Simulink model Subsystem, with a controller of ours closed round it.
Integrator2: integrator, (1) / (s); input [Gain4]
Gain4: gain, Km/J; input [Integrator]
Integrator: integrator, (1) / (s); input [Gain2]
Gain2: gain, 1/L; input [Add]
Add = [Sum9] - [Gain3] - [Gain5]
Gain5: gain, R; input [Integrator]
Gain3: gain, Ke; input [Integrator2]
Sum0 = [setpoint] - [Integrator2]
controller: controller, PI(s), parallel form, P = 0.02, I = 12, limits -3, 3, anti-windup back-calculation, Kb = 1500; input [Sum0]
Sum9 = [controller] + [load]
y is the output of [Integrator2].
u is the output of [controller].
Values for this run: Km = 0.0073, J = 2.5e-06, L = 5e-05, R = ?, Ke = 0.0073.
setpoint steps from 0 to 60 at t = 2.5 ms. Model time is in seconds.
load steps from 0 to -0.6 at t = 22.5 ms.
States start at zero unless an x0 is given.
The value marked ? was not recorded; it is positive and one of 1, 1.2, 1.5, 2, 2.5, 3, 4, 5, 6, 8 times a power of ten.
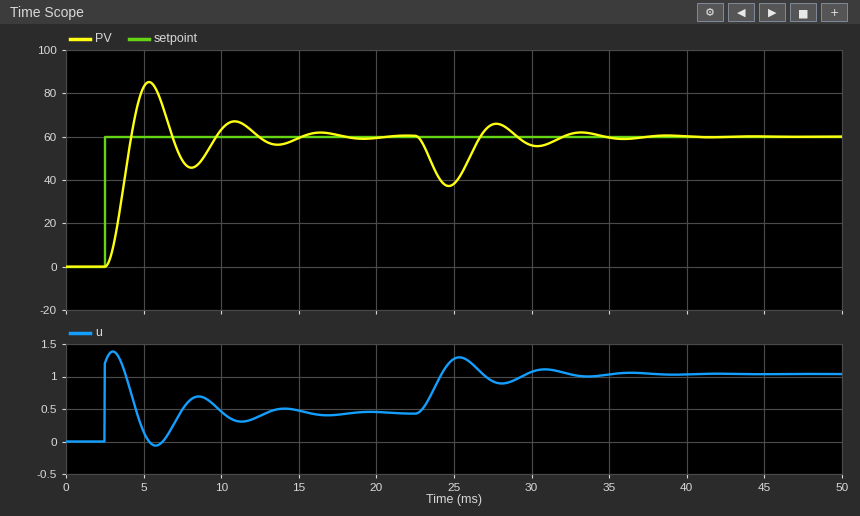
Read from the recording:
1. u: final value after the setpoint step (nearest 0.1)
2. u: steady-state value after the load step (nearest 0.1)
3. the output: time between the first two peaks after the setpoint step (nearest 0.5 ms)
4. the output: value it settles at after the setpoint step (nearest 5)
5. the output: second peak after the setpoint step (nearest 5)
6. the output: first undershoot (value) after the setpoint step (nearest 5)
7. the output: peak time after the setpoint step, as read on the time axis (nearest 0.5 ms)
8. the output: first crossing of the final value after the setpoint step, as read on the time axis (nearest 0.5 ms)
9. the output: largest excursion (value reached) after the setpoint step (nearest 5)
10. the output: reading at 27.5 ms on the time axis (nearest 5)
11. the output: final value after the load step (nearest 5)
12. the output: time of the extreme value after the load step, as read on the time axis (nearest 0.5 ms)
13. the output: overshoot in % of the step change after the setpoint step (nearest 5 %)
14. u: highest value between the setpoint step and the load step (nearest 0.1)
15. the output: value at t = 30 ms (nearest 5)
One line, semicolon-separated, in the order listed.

0.4; 1.0; 5.5 ms; 60; 65; 45; 5.5 ms; 4.0 ms; 85; 65; 60; 24.5 ms; 40 %; 1.4; 55
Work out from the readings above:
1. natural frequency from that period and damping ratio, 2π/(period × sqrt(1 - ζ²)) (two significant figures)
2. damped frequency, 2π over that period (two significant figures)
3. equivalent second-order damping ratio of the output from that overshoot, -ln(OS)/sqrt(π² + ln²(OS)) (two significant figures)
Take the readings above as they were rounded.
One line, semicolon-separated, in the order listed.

1.2 rad/ms; 1.1 rad/ms; 0.28
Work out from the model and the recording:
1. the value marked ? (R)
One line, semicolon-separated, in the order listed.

0.05
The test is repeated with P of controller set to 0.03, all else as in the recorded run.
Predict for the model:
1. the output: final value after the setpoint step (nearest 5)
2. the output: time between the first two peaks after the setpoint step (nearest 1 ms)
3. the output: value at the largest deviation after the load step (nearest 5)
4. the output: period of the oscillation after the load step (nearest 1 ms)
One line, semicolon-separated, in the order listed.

60; 5 ms; 40; 5 ms
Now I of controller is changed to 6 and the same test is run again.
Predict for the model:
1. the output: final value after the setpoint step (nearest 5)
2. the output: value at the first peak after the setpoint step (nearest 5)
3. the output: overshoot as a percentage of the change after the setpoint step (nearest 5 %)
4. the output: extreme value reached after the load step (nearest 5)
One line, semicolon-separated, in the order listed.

60; 70; 20 %; 35
